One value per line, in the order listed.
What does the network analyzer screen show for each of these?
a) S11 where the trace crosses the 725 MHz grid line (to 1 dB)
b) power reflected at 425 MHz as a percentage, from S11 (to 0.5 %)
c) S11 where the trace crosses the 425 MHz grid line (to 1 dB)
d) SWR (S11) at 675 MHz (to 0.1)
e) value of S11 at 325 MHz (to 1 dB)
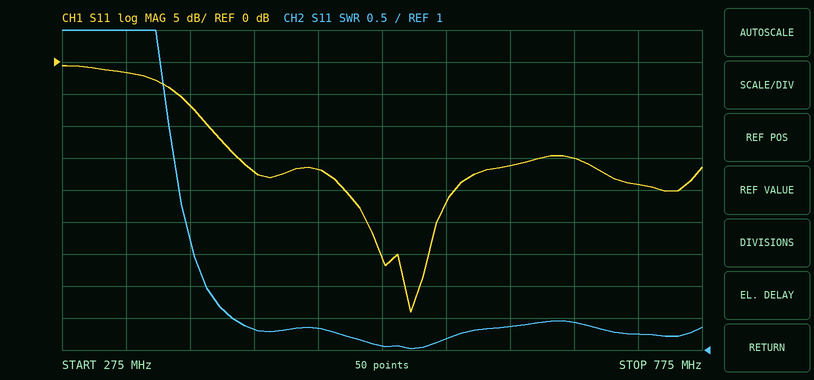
-19 dB
2.0 %
-17 dB
1.4
-2 dB
